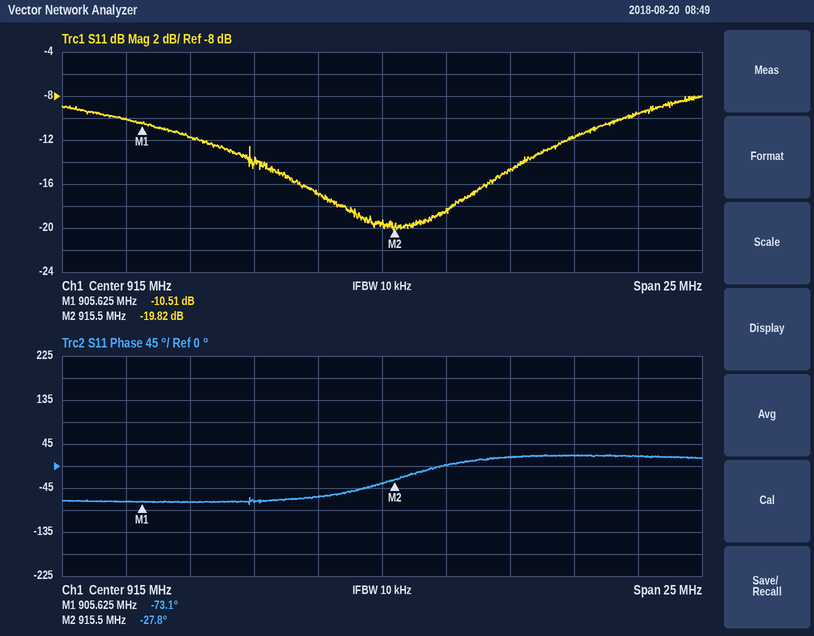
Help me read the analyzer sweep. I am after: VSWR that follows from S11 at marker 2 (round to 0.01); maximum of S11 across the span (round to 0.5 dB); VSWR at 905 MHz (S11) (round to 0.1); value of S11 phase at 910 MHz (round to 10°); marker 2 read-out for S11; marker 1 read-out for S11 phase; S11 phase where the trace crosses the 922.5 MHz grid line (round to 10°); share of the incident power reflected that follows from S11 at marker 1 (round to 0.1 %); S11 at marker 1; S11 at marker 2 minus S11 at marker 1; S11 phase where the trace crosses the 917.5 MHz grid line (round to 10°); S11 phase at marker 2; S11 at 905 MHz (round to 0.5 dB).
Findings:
1.23
-8.0 dB
1.9
-70°
-19.82 dB
-73.1°
20°
8.9 %
-10.51 dB
-9.31 dB
0°
-27.8°
-10.0 dB
